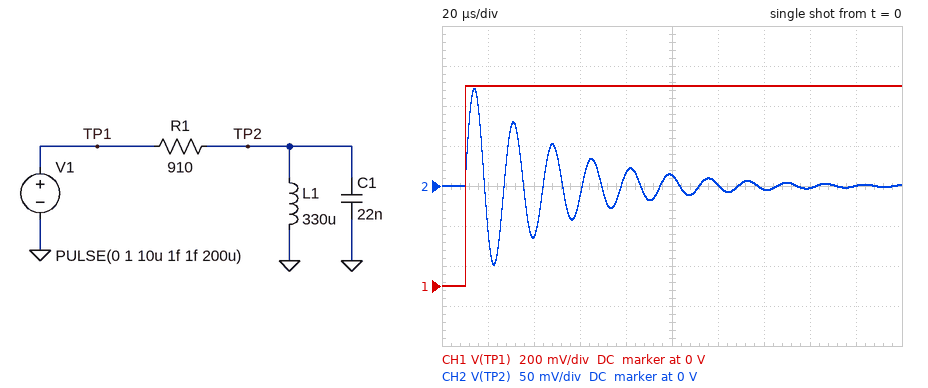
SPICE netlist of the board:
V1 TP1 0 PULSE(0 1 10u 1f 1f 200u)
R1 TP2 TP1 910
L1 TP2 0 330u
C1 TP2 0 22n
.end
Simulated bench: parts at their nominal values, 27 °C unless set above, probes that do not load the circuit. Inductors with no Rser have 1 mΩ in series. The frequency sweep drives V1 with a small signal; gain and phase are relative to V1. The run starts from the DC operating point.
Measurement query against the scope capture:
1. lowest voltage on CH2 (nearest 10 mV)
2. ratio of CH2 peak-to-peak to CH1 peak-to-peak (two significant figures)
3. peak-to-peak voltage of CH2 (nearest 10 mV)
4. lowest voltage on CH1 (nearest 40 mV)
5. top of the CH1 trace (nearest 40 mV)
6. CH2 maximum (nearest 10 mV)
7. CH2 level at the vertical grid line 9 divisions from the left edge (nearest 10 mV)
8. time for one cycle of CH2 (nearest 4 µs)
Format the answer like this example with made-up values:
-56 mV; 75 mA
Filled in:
-100 mV; 0.22; 220 mV; 0 V; 1.00 V; 120 mV; 0 V; 16 µs
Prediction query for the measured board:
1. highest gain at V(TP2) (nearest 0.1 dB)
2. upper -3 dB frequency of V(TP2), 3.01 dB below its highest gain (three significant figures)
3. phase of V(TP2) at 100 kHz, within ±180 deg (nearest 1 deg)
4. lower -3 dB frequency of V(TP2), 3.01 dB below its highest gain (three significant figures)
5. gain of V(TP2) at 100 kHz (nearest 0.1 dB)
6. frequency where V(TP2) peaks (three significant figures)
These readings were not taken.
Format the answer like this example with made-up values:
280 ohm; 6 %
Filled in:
0 dB; 63.2 kHz; -83 deg; 55.2 kHz; -18.3 dB; 59.1 kHz
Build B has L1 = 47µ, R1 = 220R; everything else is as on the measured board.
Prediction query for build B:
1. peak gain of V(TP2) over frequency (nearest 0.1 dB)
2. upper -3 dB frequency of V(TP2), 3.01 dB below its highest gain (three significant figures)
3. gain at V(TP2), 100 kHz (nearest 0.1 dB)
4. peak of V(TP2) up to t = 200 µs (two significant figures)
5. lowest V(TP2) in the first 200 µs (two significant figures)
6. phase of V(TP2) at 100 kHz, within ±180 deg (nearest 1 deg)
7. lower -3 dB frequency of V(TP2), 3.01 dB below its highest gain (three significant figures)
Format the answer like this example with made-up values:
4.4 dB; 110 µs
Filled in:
0 dB; 174 kHz; -13.1 dB; 180 mV; -130 mV; 77 deg; 141 kHz
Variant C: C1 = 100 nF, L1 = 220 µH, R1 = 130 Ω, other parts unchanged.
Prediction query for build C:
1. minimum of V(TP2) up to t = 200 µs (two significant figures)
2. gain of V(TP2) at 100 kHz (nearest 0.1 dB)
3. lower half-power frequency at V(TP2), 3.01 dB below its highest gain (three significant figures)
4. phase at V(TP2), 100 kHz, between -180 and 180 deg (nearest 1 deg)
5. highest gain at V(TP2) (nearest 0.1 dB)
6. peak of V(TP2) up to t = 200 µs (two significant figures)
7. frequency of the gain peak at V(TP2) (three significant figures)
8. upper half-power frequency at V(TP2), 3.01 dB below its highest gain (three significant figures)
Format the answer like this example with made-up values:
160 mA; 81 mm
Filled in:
-160 mV; -17.3 dB; 28.4 kHz; -82 deg; 0 dB; 280 mV; 33.9 kHz; 40.6 kHz
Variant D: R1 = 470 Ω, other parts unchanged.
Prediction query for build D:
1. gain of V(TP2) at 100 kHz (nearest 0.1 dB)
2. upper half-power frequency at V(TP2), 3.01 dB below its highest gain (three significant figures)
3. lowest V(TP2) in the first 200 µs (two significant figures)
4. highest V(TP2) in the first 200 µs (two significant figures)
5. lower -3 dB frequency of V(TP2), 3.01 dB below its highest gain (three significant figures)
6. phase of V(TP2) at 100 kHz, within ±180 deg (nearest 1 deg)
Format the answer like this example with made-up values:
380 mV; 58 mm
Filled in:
-12.8 dB; 67.3 kHz; -140 mV; 220 mV; 51.9 kHz; -77 deg
